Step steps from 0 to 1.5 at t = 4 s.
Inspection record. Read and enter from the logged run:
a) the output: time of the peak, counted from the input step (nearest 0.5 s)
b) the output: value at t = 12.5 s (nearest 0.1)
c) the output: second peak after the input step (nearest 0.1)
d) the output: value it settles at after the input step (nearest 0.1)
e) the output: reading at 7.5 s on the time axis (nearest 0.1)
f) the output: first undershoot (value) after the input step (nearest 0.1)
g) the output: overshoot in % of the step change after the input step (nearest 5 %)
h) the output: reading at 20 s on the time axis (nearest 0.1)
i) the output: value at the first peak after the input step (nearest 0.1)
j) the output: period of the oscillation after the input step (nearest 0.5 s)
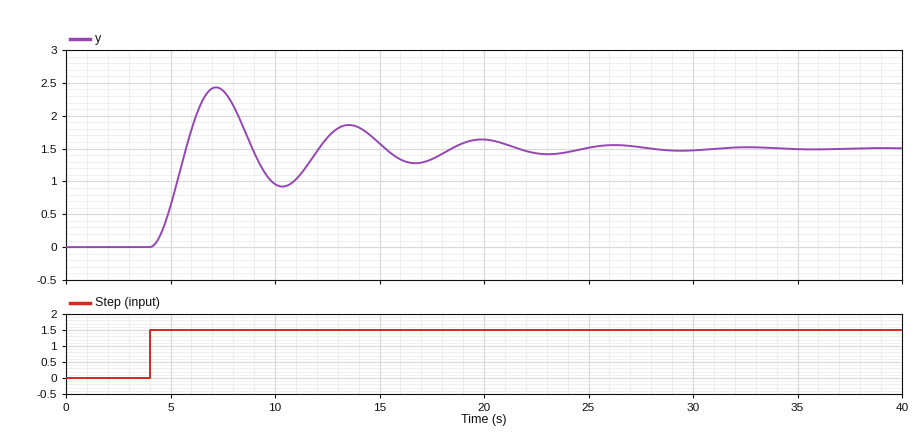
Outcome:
3.0 s
1.7
1.9
1.5
2.4
0.9
60 %
1.6
2.4
6.5 s
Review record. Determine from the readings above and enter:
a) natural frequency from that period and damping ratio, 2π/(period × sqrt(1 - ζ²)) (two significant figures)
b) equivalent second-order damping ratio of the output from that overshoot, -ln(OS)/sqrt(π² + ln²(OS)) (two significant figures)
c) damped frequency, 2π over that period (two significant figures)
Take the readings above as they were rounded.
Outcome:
0.98 rad/s
0.16
0.97 rad/s
